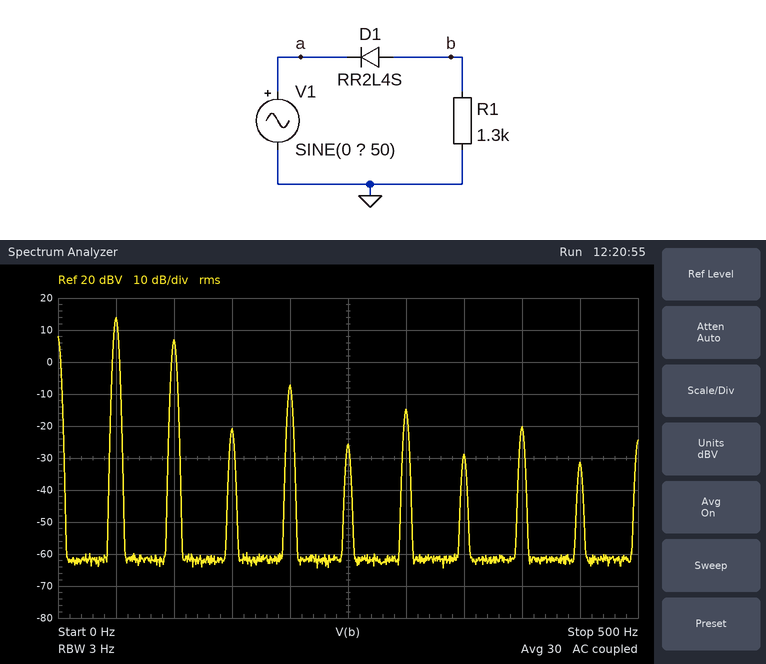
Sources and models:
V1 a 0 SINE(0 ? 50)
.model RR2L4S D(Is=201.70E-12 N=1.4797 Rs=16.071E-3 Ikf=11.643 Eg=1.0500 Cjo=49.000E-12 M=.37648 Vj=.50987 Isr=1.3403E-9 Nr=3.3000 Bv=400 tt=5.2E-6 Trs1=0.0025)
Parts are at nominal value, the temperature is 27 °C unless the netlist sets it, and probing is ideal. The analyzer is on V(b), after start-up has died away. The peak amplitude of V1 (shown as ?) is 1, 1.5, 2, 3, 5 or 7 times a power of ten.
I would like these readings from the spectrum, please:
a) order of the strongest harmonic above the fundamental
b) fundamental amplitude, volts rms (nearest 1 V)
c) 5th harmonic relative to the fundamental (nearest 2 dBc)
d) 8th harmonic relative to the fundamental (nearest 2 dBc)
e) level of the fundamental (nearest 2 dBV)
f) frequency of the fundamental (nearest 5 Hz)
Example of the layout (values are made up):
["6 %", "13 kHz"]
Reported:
["2", "5 V", "-40 dBc", "-34 dBc", "14 dBV", "50 Hz"]
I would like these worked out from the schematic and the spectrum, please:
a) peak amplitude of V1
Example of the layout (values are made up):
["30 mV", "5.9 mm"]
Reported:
["15 V"]
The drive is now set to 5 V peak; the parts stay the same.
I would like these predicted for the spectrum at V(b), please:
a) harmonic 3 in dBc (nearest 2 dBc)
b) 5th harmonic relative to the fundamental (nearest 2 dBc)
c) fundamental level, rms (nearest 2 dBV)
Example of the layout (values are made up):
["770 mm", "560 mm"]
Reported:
["-26 dBc", "-30 dBc", "4 dBV"]
